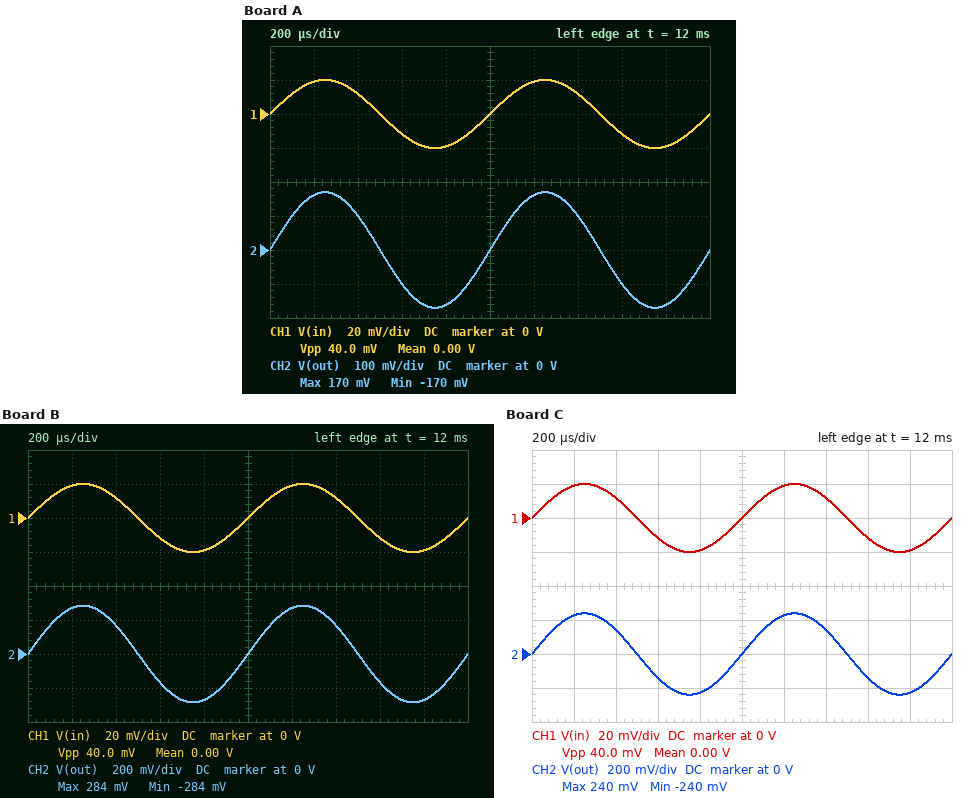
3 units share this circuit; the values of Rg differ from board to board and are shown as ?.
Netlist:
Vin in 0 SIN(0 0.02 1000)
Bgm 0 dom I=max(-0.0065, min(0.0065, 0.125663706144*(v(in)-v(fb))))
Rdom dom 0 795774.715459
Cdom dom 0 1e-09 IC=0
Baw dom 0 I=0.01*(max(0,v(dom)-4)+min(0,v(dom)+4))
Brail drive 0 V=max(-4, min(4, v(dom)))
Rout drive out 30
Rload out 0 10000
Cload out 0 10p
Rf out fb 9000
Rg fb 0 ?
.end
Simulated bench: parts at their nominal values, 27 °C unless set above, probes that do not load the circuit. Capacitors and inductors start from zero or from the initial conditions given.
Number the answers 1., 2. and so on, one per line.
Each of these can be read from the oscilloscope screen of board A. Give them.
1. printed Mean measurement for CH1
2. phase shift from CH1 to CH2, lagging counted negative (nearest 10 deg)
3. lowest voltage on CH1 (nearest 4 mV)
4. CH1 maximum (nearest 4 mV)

1. 0.00 V
2. 0 deg
3. -20 mV
4. 20 mV
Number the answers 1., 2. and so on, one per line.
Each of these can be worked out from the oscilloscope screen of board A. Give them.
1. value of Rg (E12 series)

1. 1.2 kΩ
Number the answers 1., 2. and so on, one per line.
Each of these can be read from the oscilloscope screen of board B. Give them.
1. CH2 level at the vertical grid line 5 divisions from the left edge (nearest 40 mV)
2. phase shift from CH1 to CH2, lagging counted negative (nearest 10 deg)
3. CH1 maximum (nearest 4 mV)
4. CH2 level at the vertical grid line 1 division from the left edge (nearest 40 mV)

1. 0 V
2. 0 deg
3. 20 mV
4. 280 mV
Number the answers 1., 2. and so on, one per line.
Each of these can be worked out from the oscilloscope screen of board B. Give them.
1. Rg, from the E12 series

1. 680 Ω
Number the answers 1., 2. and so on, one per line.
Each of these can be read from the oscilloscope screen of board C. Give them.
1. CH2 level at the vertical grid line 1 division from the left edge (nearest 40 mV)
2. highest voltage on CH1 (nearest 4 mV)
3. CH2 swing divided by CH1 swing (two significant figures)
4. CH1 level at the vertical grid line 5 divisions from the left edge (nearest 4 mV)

1. 240 mV
2. 20 mV
3. 12
4. 0 V
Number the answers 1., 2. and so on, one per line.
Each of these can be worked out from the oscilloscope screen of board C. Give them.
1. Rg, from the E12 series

1. 820 Ω
